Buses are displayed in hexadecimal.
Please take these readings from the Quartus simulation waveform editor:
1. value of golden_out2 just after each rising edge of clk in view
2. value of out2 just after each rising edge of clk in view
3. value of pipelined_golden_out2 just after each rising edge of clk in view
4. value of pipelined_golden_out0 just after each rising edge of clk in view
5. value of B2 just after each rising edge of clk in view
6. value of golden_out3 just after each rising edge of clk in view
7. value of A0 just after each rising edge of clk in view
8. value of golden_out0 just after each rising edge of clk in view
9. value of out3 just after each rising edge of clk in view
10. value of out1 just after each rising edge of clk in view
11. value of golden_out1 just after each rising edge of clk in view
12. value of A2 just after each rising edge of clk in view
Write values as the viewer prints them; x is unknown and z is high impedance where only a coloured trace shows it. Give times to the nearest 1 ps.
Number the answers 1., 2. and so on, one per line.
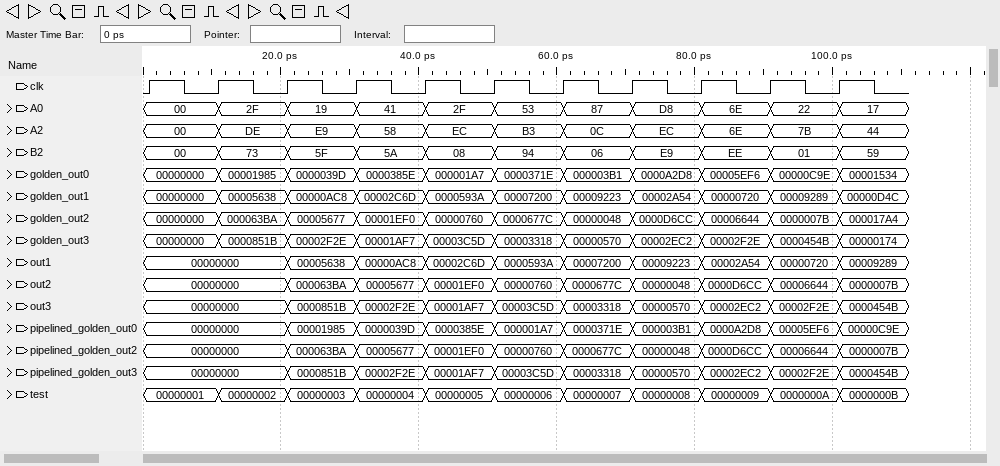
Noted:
1. 00000000, 000063BA, 00005677, 00001EF0, 00000760, 0000677C, 00000048, 0000D6CC, 00006644, 0000007B, 000017A4
2. 00000000, 00000000, 000063BA, 00005677, 00001EF0, 00000760, 0000677C, 00000048, 0000D6CC, 00006644, 0000007B
3. 00000000, 00000000, 000063BA, 00005677, 00001EF0, 00000760, 0000677C, 00000048, 0000D6CC, 00006644, 0000007B
4. 00000000, 00000000, 00001985, 0000039D, 0000385E, 000001A7, 0000371E, 000003B1, 0000A2D8, 00005EF6, 00000C9E
5. 00, 73, 5F, 5A, 08, 94, 06, E9, EE, 01, 59
6. 00000000, 0000851B, 00002F2E, 00001AF7, 00003C5D, 00003318, 00000570, 00002EC2, 00002F2E, 0000454B, 00000174
7. 00, 2F, 19, 41, 2F, 53, 87, D8, 6E, 22, 17
8. 00000000, 00001985, 0000039D, 0000385E, 000001A7, 0000371E, 000003B1, 0000A2D8, 00005EF6, 00000C9E, 00001534
9. 00000000, 00000000, 0000851B, 00002F2E, 00001AF7, 00003C5D, 00003318, 00000570, 00002EC2, 00002F2E, 0000454B
10. 00000000, 00000000, 00005638, 00000AC8, 00002C6D, 0000593A, 00007200, 00009223, 00002A54, 00000720, 00009289
11. 00000000, 00005638, 00000AC8, 00002C6D, 0000593A, 00007200, 00009223, 00002A54, 00000720, 00009289, 00000D4C
12. 00, DE, E9, 58, EC, B3, 0C, EC, 6E, 7B, 44
